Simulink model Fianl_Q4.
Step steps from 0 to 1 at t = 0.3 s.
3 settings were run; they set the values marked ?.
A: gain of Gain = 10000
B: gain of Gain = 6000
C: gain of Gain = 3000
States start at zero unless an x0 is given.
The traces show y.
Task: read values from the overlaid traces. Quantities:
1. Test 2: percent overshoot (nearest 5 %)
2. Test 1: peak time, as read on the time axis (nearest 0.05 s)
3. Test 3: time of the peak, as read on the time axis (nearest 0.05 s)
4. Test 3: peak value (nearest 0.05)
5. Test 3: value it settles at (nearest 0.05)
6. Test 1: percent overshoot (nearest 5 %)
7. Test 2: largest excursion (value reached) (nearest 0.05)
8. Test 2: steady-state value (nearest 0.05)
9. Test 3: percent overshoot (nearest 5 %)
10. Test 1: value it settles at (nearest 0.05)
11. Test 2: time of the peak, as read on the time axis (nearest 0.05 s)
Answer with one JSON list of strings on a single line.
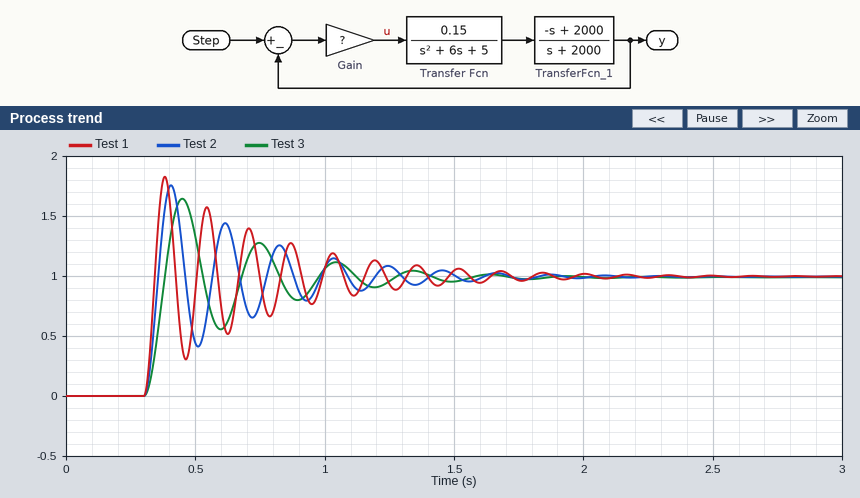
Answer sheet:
["75 %", "0.40 s", "0.45 s", "1.65", "1.00", "85 %", "1.75", "1.00", "65 %", "1.00", "0.40 s"]
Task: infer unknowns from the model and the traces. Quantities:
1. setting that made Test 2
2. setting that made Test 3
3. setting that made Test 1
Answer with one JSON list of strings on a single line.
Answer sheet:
["B", "C", "A"]
